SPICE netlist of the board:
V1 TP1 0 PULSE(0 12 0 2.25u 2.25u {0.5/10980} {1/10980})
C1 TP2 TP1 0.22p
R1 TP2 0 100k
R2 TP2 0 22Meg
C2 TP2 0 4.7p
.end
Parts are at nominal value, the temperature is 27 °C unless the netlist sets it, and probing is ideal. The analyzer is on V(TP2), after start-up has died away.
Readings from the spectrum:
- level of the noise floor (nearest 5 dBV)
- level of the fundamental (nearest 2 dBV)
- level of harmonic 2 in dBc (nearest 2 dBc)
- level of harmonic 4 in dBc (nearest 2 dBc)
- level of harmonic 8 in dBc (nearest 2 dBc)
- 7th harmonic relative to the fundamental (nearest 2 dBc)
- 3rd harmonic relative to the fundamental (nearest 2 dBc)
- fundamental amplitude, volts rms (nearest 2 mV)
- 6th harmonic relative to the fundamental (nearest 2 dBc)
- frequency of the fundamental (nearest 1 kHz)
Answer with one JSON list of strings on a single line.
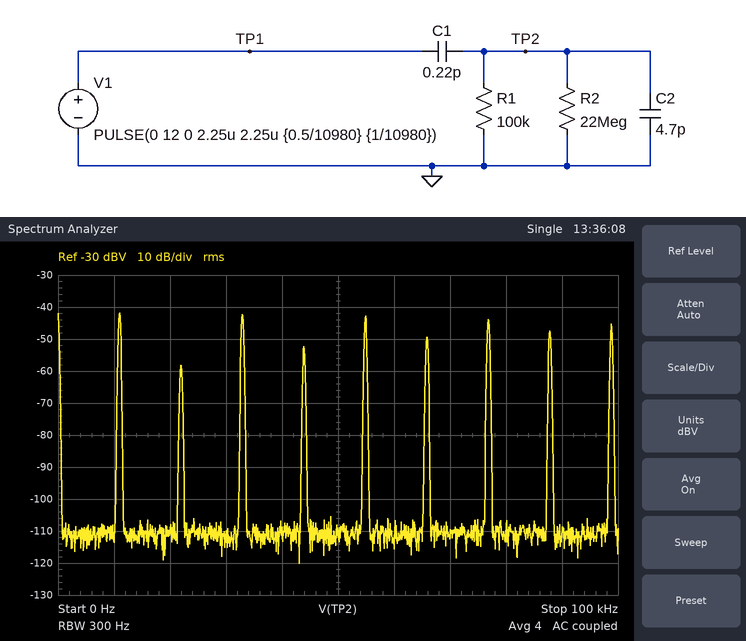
["-110 dBV", "-42 dBV", "-16 dBc", "-10 dBc", "-6 dBc", "-2 dBc", "0 dBc", "8 mV", "-8 dBc", "11 kHz"]
